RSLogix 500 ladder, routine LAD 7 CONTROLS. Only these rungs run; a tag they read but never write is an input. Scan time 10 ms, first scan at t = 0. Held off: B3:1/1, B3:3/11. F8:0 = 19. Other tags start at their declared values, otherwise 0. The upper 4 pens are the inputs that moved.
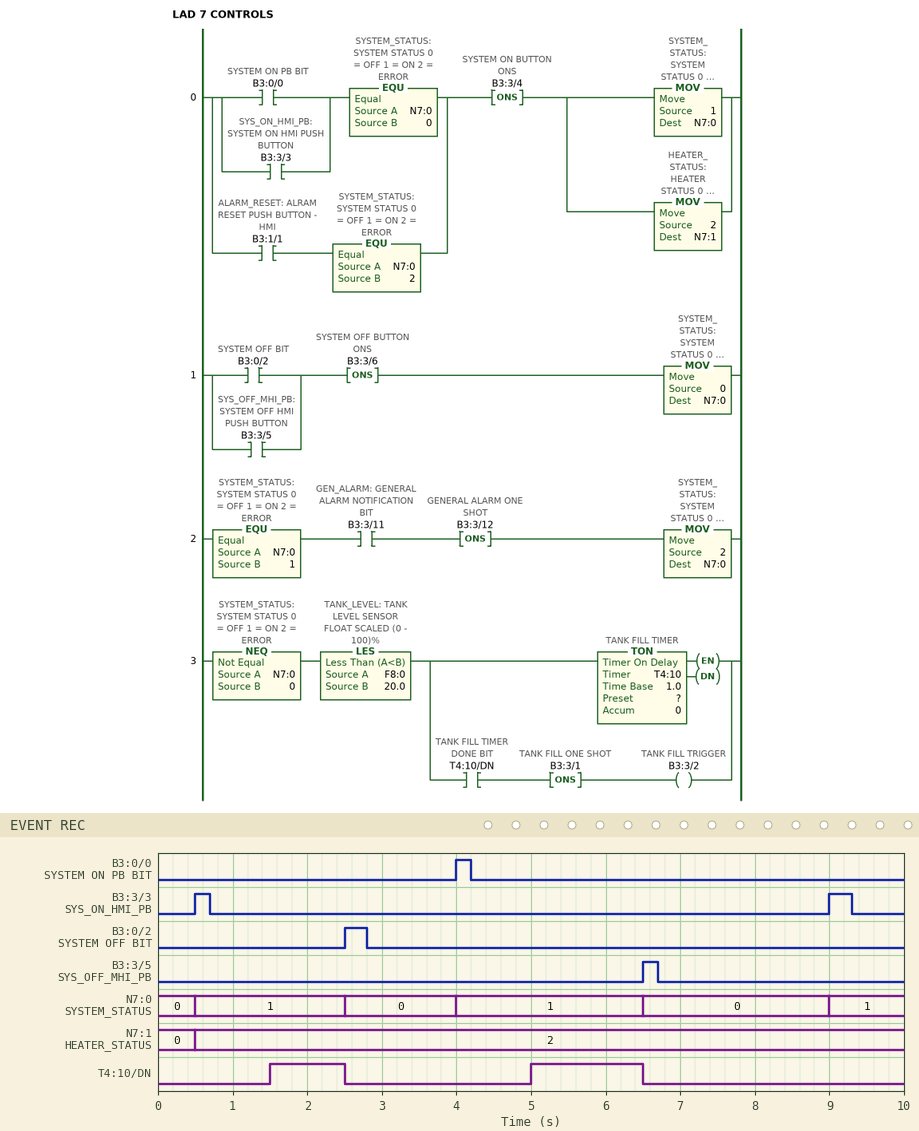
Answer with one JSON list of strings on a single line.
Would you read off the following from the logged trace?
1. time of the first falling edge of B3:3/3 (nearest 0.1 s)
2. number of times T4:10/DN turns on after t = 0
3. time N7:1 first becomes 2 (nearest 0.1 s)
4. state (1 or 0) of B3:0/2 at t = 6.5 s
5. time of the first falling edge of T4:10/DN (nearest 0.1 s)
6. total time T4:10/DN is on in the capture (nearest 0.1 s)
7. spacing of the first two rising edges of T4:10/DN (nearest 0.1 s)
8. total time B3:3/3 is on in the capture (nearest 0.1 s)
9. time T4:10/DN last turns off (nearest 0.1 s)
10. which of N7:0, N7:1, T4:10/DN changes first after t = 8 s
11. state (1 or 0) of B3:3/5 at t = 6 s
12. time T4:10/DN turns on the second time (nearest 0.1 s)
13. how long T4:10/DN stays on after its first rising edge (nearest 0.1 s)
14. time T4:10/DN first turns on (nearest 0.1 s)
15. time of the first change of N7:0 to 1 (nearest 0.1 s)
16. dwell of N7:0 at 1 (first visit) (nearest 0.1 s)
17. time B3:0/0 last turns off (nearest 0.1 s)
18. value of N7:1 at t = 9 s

["0.7 s", "2", "0.5 s", "0", "2.5 s", "2.5 s", "3.5 s", "0.5 s", "6.5 s", "N7:0", "0", "5.0 s", "1.0 s", "1.5 s", "0.5 s", "2.0 s", "4.2 s", "2"]
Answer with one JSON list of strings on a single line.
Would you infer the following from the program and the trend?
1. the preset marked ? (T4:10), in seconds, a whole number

["1 s"]
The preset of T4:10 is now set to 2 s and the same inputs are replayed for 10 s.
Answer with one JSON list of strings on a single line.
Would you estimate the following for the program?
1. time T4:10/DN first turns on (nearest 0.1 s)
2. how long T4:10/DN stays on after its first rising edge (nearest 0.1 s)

["6.0 s", "0.5 s"]
